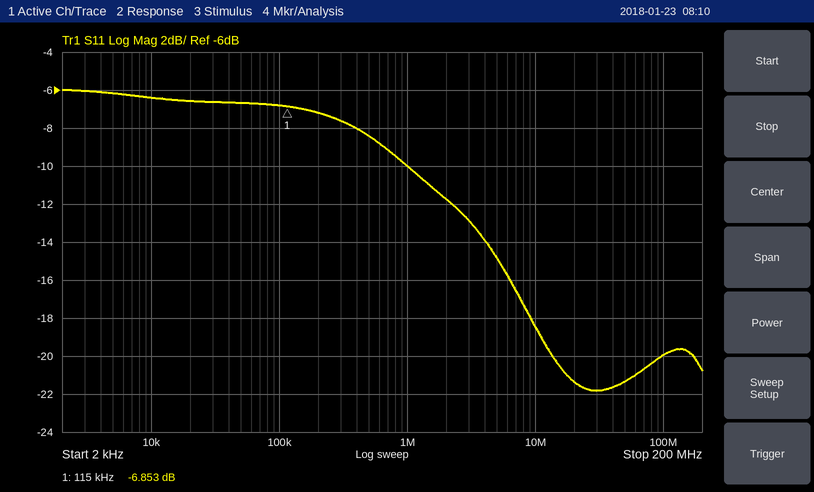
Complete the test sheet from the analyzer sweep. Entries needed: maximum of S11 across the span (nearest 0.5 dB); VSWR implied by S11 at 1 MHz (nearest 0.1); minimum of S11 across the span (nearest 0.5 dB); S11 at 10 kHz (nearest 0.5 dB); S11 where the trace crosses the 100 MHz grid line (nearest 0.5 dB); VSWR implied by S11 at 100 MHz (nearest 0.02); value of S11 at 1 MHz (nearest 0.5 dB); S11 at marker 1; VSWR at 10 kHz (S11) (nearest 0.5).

-6.0 dB
1.9
-22.0 dB
-6.5 dB
-20.0 dB
1.22
-10.0 dB
-6.853 dB
3.0
